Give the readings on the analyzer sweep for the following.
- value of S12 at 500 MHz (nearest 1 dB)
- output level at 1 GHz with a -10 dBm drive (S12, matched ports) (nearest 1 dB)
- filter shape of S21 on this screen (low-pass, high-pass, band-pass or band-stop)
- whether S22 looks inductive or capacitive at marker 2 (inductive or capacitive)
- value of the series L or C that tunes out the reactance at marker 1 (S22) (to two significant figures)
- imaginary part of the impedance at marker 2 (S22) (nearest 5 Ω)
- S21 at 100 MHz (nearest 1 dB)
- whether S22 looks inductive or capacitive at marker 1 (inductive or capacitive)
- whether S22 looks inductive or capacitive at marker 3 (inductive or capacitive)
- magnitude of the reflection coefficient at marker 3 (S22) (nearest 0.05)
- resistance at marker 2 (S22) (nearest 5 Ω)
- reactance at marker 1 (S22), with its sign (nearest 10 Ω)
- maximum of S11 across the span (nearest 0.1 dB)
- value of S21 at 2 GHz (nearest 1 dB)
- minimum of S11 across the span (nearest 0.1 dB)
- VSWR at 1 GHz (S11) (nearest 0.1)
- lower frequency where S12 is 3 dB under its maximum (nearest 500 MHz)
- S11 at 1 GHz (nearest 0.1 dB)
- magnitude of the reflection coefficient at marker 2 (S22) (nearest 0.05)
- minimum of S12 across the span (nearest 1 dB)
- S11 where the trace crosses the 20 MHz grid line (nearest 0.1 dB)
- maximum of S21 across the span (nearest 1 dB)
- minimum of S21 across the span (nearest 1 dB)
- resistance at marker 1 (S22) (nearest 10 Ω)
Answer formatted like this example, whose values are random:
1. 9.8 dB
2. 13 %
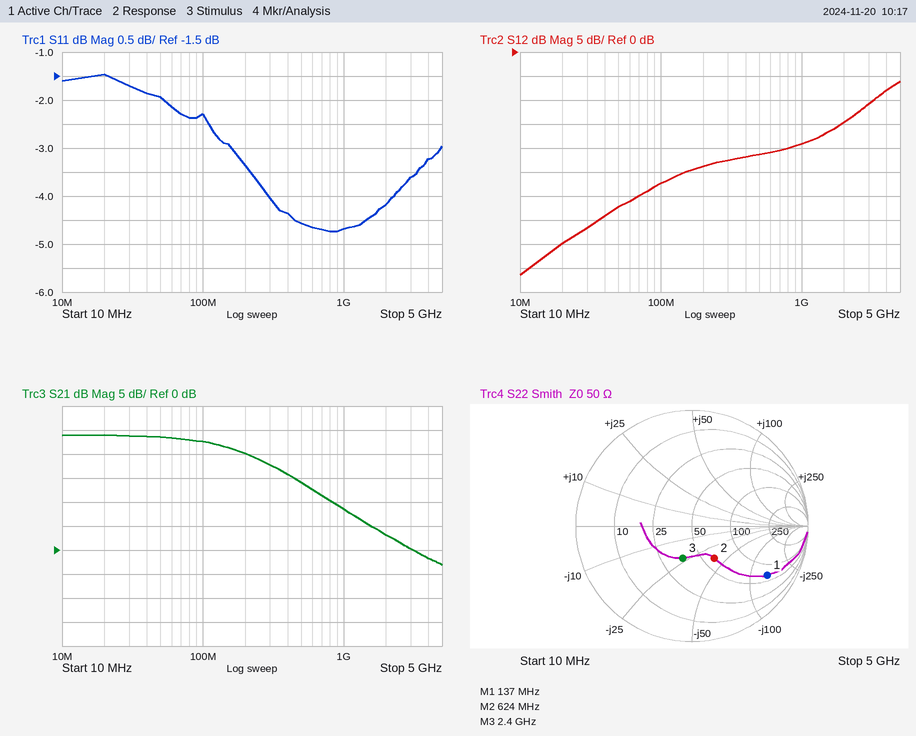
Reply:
1. -21 dB
2. -29 dBm
3. low-pass
4. capacitive
5. 160 nH
6. -40 Ω
7. 23 dB
8. capacitive
9. capacitive
10. 0.30
11. 60 Ω
12. -140 Ω
13. -1.5 dB
14. 3 dB
15. -4.7 dB
16. 3.8
17. 3.5 GHz
18. -4.7 dB
19. 0.35
20. -46 dB
21. -1.5 dB
22. 24 dB
23. -3 dB
24. 70 Ω
